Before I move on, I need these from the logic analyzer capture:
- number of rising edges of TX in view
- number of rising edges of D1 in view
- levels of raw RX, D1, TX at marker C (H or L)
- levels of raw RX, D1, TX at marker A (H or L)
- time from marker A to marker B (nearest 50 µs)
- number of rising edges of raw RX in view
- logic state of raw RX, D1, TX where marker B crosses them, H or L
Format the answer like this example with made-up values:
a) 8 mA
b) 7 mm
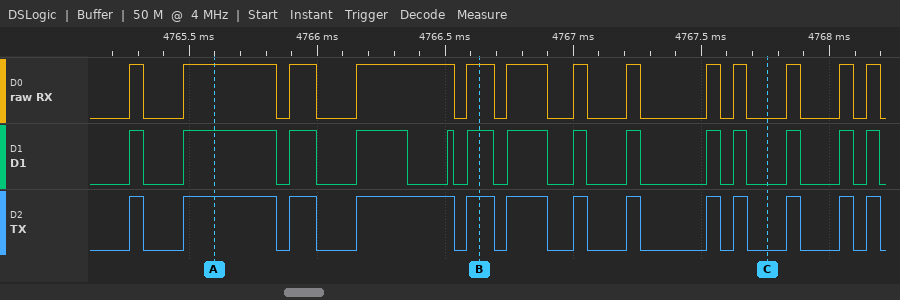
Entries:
a) 13
b) 14
c) raw RX=L, D1=L, TX=L
d) raw RX=H, D1=H, TX=H
e) 1050 µs
f) 13
g) raw RX=H, D1=H, TX=H
